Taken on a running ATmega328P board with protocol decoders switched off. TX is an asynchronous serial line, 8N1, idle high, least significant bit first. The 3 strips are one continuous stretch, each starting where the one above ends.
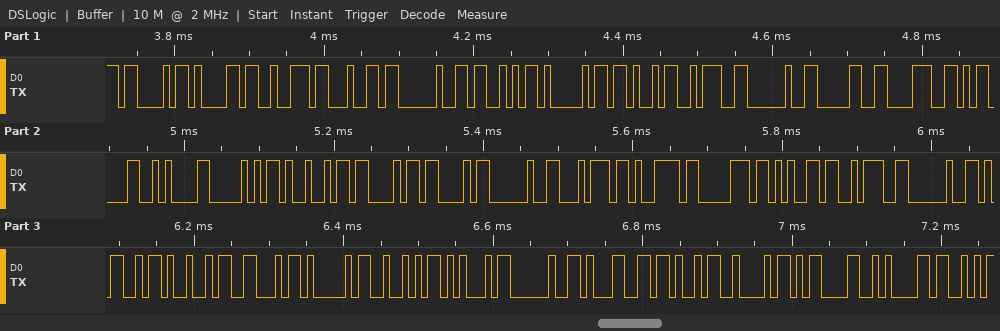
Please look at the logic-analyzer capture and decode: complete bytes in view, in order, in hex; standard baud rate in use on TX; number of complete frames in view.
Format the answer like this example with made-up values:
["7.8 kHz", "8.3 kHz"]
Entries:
["0x43 0x61 0x72 0x64 0x20 0x53 0x41 0x4B 0x3A 0x20 0x30 0x38 0x0D 0x0A 0x50 0x49 0x43 0x43 0x20 0x74 0x79 0x70 0x65 0x3A 0x20 0x4D 0x49 0x46 0x41 0x52 0x45 0x20 0x31 0x4B 0x42 0x0D 0x0A 0x53", "115200 baud", "38"]
